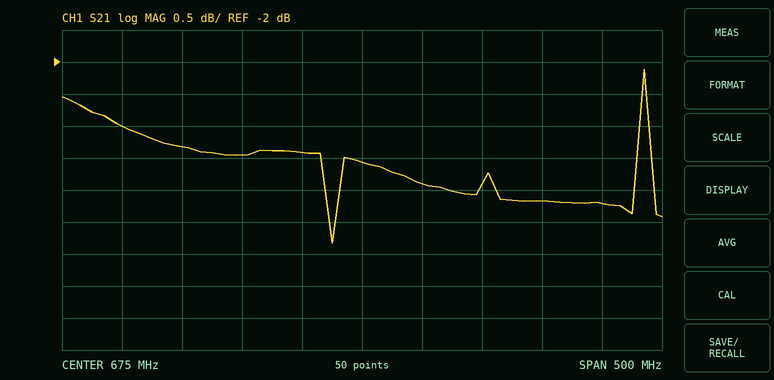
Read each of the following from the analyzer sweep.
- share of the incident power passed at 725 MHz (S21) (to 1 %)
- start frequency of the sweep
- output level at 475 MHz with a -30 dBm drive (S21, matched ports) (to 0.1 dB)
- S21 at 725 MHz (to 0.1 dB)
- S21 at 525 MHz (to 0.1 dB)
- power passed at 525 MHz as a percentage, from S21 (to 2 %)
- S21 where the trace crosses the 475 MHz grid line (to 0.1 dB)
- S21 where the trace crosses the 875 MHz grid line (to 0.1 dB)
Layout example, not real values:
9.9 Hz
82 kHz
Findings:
41 %
425 MHz
-33.0 dBm
-3.9 dB
-3.3 dB
46 %
-3.0 dB
-4.2 dB
